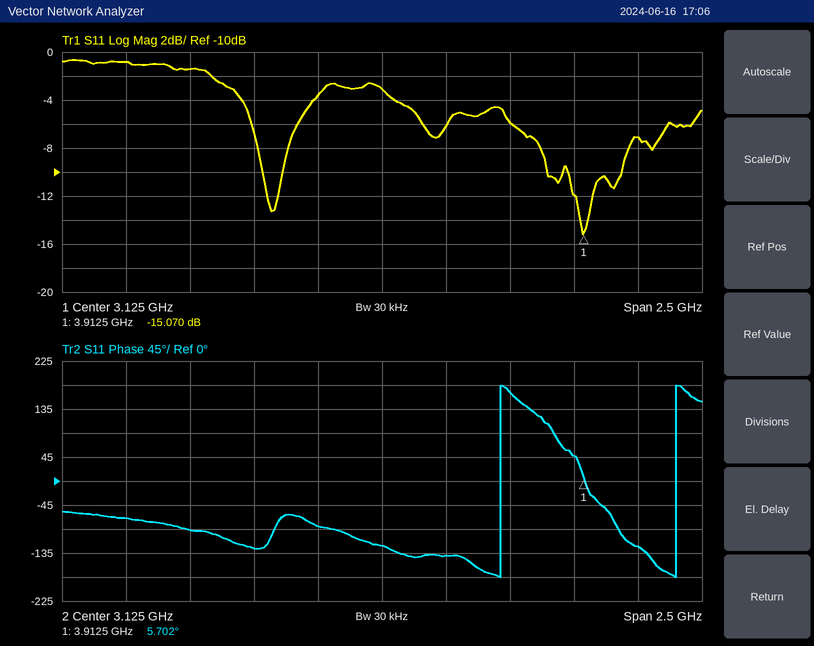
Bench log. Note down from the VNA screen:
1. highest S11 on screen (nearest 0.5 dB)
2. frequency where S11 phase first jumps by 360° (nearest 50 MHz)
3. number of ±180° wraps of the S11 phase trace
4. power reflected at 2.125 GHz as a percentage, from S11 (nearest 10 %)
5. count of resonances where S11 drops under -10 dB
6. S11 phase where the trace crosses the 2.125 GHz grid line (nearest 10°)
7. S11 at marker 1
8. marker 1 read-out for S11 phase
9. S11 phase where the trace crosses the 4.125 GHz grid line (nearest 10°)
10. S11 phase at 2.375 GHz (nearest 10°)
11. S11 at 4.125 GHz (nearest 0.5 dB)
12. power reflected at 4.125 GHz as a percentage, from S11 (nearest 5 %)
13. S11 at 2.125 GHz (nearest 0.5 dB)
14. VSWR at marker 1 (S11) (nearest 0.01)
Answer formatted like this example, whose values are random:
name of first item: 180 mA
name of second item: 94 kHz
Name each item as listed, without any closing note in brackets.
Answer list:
highest S11 on screen: -0.5 dB
frequency where S11 phase first jumps by 360°: 3.60 GHz
number of ±180° wraps of the S11 phase trace: 2
power reflected at 2.125 GHz as a percentage, from S11: 80 %
count of resonances where S11 drops under -10 dB: 2
S11 phase where the trace crosses the 2.125 GHz grid line: -70°
S11 at marker 1: -15.070 dB
marker 1 read-out for S11 phase: 5.702°
S11 phase where the trace crosses the 4.125 GHz grid line: -120°
S11 phase at 2.375 GHz: -90°
S11 at 4.125 GHz: -7.0 dB
power reflected at 4.125 GHz as a percentage, from S11: 20 %
S11 at 2.125 GHz: -1.0 dB
VSWR at marker 1 (S11): 1.43
